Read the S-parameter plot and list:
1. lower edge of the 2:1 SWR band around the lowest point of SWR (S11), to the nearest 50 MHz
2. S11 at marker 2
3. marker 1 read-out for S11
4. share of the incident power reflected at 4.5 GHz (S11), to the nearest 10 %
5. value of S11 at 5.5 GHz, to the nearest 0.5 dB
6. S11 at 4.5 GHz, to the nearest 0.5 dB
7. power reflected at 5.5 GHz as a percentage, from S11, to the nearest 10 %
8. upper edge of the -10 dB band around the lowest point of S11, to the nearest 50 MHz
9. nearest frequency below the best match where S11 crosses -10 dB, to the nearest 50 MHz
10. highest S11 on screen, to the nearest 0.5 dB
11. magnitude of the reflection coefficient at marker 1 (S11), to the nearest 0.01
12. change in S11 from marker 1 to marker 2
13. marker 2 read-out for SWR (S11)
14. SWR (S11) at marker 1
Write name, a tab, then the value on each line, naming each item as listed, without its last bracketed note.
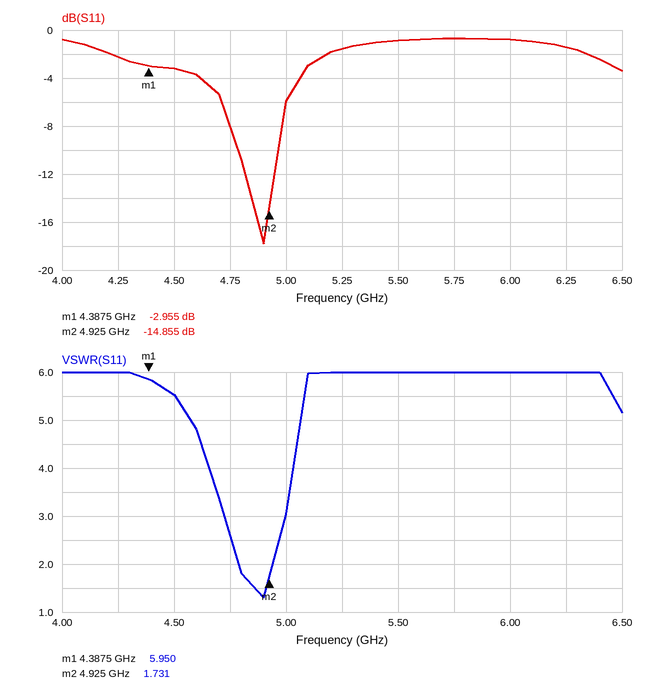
lower edge of the 2:1 SWR band around the lowest point of SWR (S11), to the nearest 50 MHz	4.80 GHz
S11 at marker 2	-14.855 dB
marker 1 read-out for S11	-2.955 dB
share of the incident power reflected at 4.5 GHz (S11), to the nearest 10 %	50 %
value of S11 at 5.5 GHz, to the nearest 0.5 dB	-1.0 dB
S11 at 4.5 GHz, to the nearest 0.5 dB	-3.0 dB
power reflected at 5.5 GHz as a percentage, from S11, to the nearest 10 %	80 %
upper edge of the -10 dB band around the lowest point of S11, to the nearest 50 MHz	4.95 GHz
nearest frequency below the best match where S11 crosses -10 dB, to the nearest 50 MHz	4.80 GHz
highest S11 on screen, to the nearest 0.5 dB	-0.5 dB
magnitude of the reflection coefficient at marker 1 (S11), to the nearest 0.01	0.71
change in S11 from marker 1 to marker 2	-11.900 dB
marker 2 read-out for SWR	1.731
SWR (S11) at marker 1	5.950
